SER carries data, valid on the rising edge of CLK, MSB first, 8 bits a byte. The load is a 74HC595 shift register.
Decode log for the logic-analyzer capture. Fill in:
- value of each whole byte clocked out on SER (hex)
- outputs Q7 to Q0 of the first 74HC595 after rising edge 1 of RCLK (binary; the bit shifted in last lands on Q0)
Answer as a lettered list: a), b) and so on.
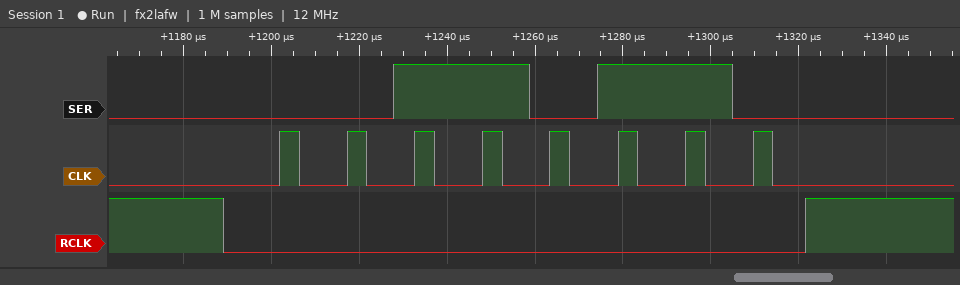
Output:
a) 36
b) 00110110
